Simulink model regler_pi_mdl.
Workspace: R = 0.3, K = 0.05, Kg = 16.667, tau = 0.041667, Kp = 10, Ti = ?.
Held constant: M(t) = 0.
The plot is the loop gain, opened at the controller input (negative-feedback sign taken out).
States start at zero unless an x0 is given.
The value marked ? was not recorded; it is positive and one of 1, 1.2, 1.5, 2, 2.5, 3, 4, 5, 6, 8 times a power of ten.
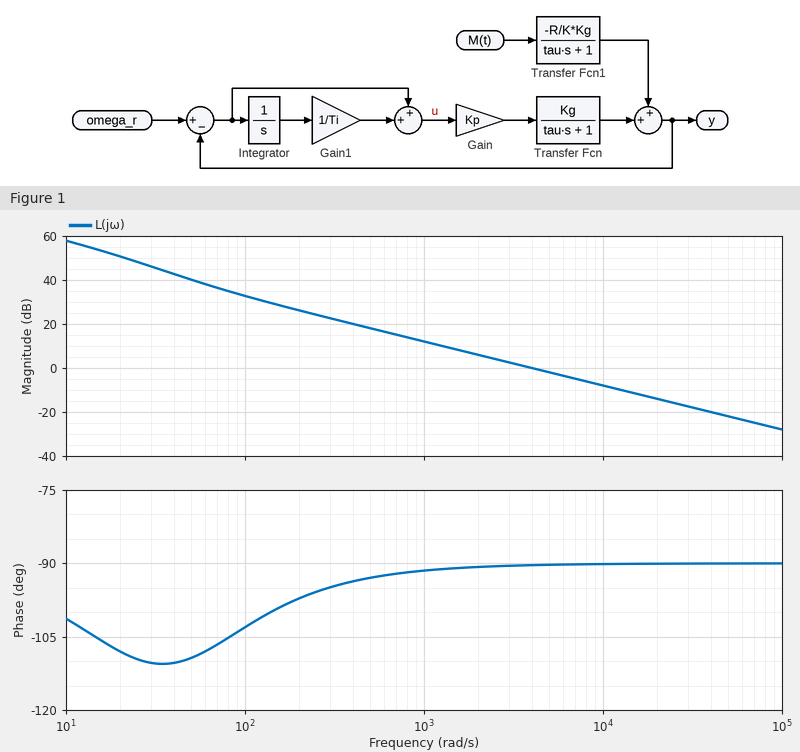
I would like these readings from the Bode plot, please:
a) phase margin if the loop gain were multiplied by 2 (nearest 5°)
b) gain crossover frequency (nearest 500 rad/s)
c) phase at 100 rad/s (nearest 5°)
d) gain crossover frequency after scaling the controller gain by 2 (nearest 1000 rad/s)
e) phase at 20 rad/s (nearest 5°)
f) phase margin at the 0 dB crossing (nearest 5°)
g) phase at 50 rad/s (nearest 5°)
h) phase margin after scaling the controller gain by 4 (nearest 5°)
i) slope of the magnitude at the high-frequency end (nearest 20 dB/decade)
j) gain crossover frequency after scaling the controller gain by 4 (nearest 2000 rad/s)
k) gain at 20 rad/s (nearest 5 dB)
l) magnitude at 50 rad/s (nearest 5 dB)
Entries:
90°
4000 rad/s
-105°
8000 rad/s
-110°
90°
-110°
90°
-20 dB/decade
16000 rad/s
50 dB
40 dB
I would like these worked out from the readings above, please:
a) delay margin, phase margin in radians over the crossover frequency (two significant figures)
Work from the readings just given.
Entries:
0.00039 s
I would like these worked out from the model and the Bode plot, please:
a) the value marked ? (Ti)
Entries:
0.02
